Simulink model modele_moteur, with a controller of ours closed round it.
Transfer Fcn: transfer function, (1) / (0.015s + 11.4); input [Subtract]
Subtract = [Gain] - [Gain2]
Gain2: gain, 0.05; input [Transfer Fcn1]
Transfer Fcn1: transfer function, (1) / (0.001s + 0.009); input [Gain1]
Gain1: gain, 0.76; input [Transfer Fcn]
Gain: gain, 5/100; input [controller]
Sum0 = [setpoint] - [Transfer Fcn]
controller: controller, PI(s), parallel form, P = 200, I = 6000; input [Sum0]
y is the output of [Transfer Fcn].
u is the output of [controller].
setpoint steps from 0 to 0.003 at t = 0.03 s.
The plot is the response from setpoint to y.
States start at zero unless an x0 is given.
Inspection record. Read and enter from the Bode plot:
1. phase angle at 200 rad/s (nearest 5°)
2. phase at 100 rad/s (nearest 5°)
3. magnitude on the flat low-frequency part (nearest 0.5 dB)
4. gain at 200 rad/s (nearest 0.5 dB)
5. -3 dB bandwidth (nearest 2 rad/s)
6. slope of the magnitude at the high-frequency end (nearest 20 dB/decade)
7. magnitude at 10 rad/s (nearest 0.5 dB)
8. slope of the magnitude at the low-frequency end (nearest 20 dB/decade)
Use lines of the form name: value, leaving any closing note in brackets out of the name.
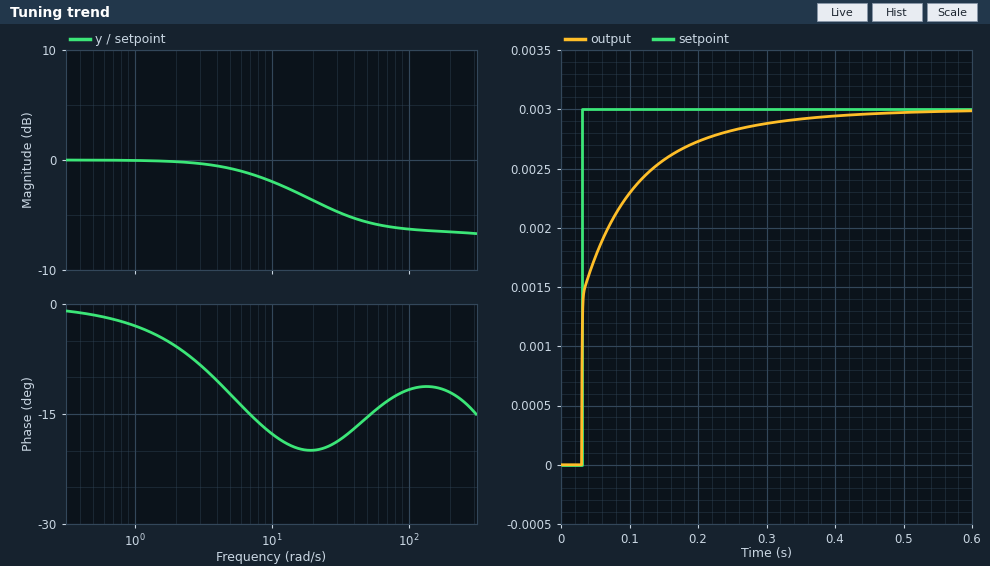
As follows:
phase angle at 200 rad/s: -10°
phase at 100 rad/s: -10°
magnitude on the flat low-frequency part: 0.0 dB
gain at 200 rad/s: -6.5 dB
-3 dB bandwidth: 16 rad/s
slope of the magnitude at the high-frequency end: 0 dB/decade
magnitude at 10 rad/s: -2.0 dB
slope of the magnitude at the low-frequency end: 0 dB/decade
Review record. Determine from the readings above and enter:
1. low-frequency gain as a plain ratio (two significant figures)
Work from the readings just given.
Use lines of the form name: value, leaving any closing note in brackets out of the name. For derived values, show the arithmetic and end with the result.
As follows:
low-frequency gain as a plain ratio: 10^(0 / 20) = 1.0
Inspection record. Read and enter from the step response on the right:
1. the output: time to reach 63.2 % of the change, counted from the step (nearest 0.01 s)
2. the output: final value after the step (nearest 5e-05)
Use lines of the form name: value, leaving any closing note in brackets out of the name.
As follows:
the output: time to reach 63.2 % of the change, counted from the step: 0.03 s
the output: final value after the step: 0.00300
